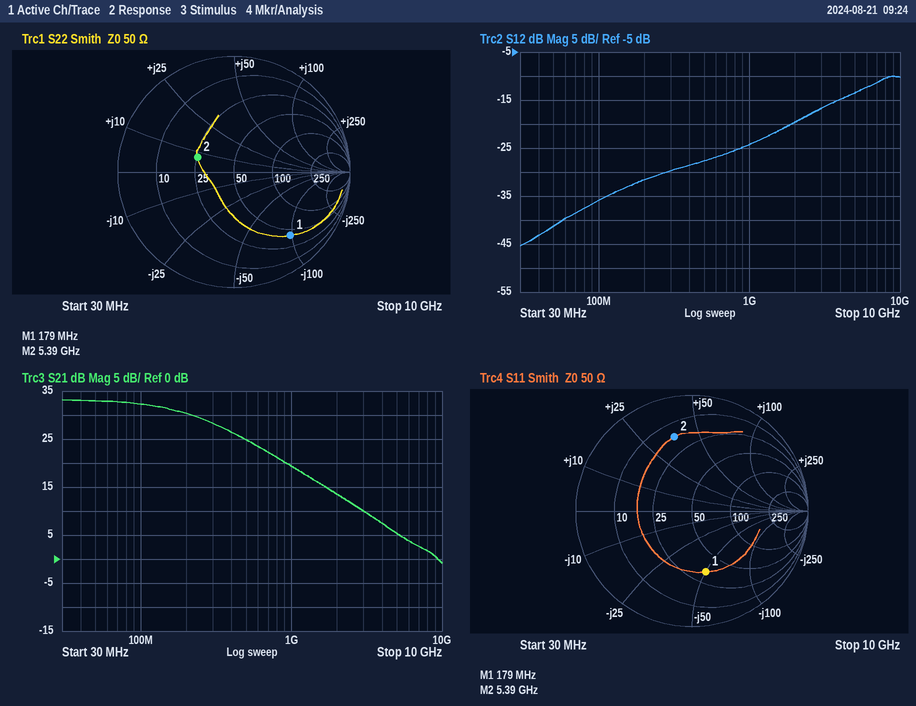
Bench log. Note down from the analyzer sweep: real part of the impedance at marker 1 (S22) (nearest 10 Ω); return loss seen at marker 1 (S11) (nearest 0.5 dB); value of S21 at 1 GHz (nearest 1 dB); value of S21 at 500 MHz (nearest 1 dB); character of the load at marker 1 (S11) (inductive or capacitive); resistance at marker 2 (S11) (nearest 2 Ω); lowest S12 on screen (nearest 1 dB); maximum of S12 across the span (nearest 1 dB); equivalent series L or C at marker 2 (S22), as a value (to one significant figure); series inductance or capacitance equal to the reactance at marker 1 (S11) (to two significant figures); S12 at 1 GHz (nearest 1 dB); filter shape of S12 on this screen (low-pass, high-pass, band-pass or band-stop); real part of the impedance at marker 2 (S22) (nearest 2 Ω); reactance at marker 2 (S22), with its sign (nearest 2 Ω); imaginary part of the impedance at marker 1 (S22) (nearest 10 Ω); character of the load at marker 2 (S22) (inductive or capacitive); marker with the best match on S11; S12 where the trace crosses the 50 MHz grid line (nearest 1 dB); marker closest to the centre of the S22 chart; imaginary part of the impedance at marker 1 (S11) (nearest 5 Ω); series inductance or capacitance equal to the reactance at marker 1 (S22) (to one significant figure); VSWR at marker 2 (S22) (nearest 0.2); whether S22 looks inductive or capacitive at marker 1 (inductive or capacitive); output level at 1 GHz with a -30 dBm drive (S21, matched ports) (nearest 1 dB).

40 Ω
5.5 dB
19 dB
25 dB
capacitive
16 Ω
-45 dB
-10 dB
200 pH
18 pF
-24 dB
high-pass
26 Ω
+8 Ω
-100 Ω
inductive
marker 1
-41 dB
marker 2
-50 Ω
9 pF
2.0
capacitive
-11 dBm
